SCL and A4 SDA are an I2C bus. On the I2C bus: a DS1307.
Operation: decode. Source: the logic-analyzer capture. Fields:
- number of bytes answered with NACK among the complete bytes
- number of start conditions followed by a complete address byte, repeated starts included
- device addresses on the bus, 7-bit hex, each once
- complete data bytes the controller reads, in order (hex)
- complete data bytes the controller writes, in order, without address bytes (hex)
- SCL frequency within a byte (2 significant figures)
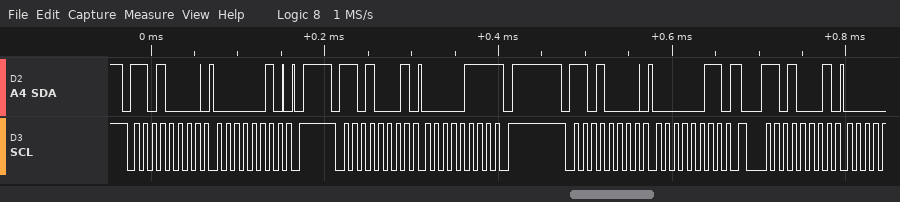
1
4
0x68
07
02 03
100 kHz
